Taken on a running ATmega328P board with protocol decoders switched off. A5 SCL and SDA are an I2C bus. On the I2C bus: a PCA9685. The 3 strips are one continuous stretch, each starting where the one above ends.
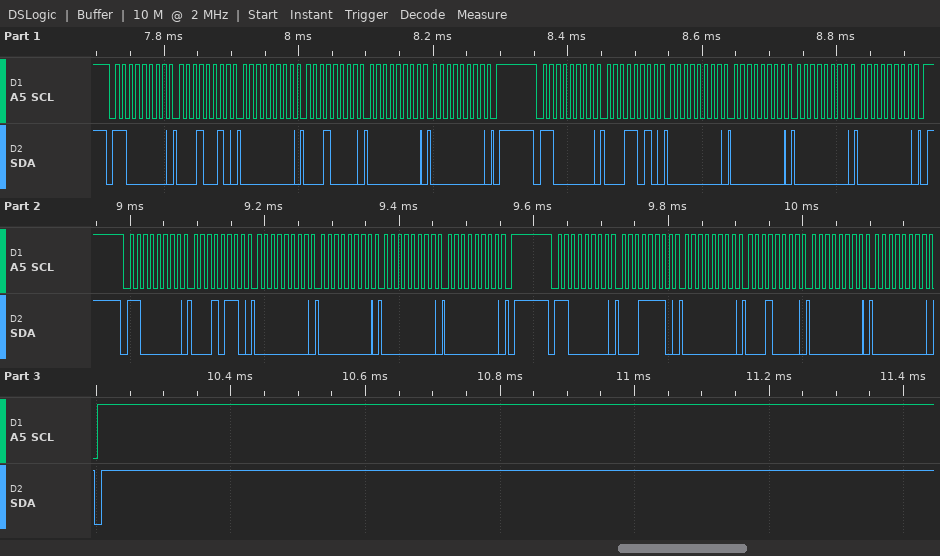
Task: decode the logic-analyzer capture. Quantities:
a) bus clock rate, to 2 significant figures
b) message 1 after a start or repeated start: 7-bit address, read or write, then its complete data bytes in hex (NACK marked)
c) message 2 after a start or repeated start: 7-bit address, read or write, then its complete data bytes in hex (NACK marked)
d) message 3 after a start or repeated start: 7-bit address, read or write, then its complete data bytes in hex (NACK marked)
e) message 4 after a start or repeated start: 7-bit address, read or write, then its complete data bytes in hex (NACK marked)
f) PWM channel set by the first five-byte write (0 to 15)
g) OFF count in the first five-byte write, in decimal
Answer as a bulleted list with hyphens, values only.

- 100 kHz
- 0x60 write: 12 00 10 00 00
- 0x60 write: 1A 00 00 00 00
- 0x60 write: 16 00 00 00 00
- 0x60 write: 1E 00 10 00 00
- 3
- 0
